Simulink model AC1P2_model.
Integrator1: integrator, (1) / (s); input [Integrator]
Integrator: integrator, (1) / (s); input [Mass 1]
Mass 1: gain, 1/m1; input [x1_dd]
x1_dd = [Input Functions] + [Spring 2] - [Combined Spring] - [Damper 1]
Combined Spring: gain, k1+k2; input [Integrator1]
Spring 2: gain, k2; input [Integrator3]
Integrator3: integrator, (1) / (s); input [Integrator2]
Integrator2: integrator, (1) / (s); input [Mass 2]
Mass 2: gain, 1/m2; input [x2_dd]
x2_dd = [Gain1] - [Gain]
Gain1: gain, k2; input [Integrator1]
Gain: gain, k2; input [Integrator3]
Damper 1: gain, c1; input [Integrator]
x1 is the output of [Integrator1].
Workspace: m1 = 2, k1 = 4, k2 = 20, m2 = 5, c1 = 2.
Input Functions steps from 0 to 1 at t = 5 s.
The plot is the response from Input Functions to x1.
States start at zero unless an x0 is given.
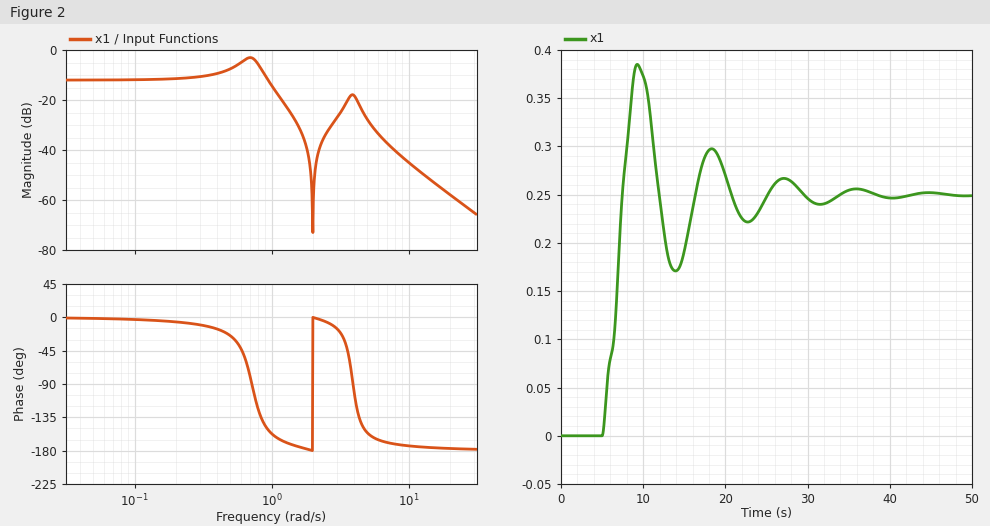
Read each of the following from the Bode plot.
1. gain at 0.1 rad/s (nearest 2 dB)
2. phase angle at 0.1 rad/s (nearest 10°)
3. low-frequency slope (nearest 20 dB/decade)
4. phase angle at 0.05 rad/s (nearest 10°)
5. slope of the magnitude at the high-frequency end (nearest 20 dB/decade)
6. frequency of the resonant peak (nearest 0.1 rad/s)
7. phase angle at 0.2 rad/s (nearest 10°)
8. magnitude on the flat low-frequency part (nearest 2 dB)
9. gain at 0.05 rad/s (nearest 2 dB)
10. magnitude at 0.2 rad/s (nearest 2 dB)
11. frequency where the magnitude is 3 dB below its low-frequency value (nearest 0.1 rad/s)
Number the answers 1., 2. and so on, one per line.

1. -12 dB
2. 0°
3. 0 dB/decade
4. 0°
5. -40 dB/decade
6. 0.7 rad/s
7. -10°
8. -12 dB
9. -12 dB
10. -12 dB
11. 1.0 rad/s
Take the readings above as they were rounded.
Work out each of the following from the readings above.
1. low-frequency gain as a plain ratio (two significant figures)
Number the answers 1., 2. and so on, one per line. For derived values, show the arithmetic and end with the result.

1. 10^(-12 / 20) = 0.25
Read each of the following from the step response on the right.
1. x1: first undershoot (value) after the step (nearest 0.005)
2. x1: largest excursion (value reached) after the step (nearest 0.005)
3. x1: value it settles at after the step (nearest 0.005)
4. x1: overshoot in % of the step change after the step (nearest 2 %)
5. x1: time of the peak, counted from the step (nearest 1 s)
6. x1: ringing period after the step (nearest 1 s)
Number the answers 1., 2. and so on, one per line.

1. 0.170
2. 0.385
3. 0.250
4. 54 %
5. 4 s
6. 9 s
